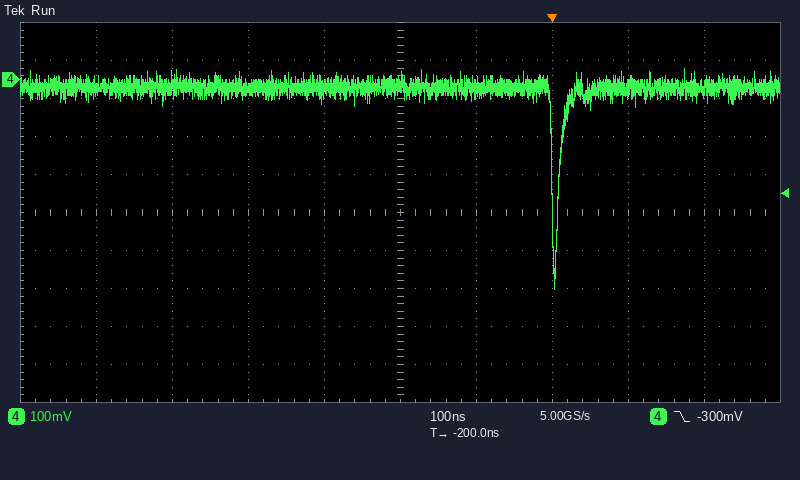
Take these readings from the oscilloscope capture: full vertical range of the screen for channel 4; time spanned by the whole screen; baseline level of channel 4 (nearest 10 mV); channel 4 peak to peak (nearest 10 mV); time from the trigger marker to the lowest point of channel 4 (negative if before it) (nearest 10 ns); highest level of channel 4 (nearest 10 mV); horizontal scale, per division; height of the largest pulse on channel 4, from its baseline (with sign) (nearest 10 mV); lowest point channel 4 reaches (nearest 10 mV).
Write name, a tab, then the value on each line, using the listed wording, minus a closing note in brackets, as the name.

full vertical range of the screen for channel 4	1 V
time spanned by the whole screen	1 µs
baseline level of channel 4	-20 mV
channel 4 peak to peak	580 mV
time from the trigger marker to the lowest point of channel 4 (negative if before it)	0 ns
highest level of channel 4	30 mV
horizontal scale, per division	100 ns
height of the largest pulse on channel 4, from its baseline (with sign)	-530 mV
lowest point channel 4 reaches	-550 mV
